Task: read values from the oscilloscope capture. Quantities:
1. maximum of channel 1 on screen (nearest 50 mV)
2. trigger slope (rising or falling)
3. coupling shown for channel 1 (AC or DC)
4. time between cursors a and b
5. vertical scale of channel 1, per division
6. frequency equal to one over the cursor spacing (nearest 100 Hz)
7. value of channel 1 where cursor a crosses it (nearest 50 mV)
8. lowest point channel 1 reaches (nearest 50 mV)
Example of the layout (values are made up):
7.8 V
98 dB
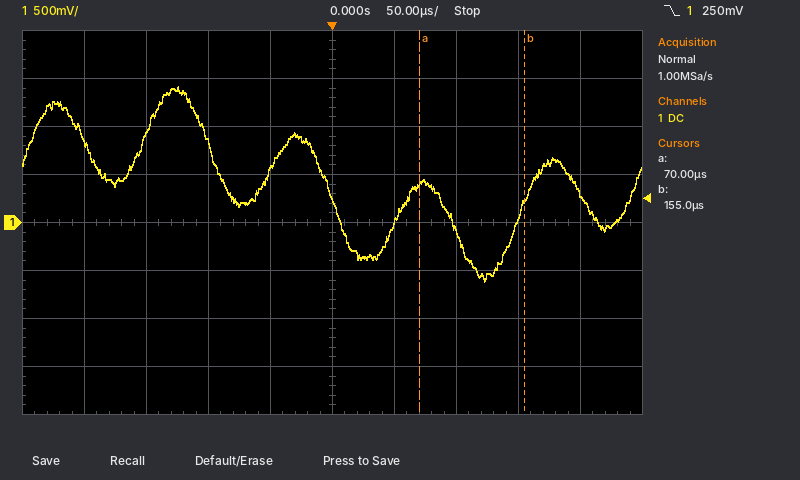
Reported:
1.40 V
falling
DC
85 µs
500 mV
11.8 kHz
400 mV
-600 mV
